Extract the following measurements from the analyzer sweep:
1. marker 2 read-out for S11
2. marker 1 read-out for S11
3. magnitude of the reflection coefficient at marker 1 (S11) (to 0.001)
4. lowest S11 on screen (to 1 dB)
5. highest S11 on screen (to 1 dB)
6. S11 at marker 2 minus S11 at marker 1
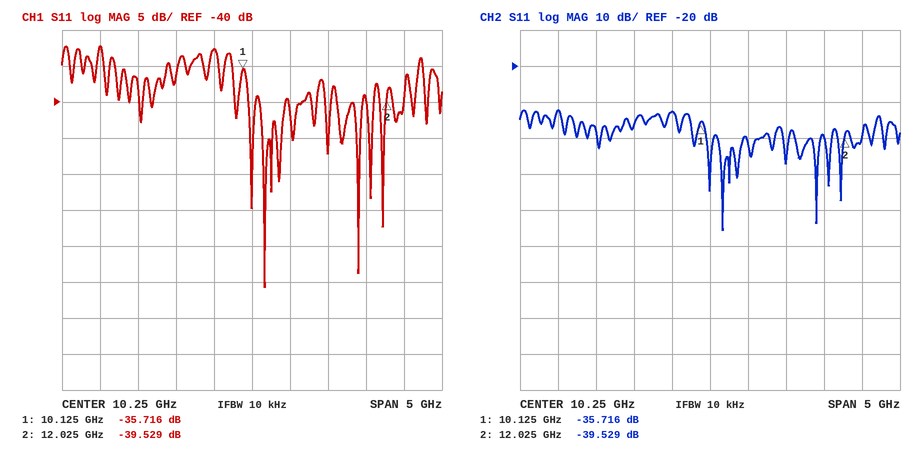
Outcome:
-39.529 dB
-35.716 dB
0.016
-66 dB
-32 dB
-3.813 dB
